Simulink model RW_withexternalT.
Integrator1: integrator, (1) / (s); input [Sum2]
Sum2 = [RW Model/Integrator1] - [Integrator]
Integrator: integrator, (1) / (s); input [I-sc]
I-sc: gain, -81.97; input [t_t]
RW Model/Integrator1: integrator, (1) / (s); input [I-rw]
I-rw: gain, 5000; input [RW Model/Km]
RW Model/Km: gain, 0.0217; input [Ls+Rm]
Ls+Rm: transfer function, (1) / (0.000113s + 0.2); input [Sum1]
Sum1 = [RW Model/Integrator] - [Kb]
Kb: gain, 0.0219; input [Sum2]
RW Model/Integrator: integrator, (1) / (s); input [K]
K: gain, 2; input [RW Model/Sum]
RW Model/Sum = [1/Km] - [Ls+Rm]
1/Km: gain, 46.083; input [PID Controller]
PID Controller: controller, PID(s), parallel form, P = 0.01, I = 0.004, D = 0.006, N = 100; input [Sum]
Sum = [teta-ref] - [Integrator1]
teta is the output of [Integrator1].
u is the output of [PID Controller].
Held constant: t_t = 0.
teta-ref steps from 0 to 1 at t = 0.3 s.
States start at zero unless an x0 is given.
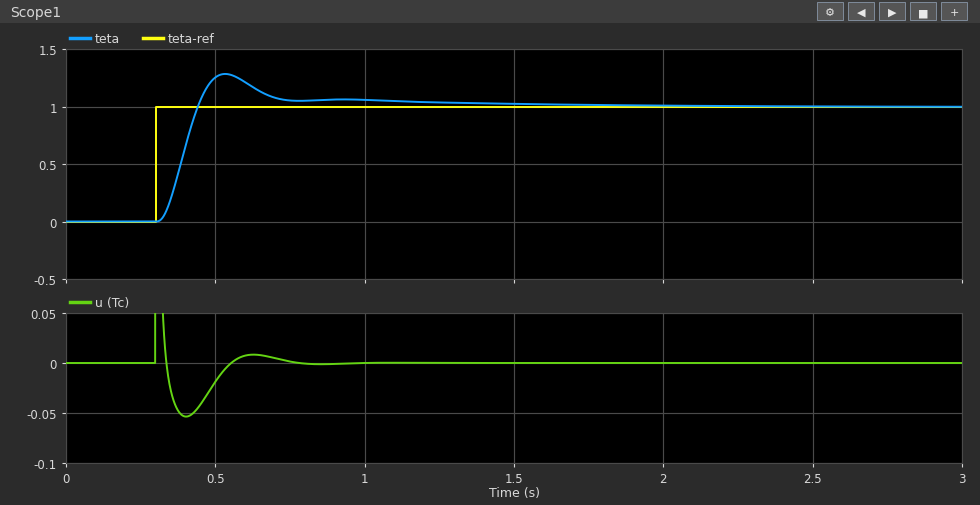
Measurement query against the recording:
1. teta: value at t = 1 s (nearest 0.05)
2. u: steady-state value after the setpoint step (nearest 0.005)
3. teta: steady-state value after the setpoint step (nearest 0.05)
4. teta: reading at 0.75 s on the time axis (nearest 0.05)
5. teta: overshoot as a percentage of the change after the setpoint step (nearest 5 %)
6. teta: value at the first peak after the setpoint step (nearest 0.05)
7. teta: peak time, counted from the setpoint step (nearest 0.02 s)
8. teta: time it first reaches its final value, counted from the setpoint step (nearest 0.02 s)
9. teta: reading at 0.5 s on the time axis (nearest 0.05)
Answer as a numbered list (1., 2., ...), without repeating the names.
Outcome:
1. 1.05
2. 0.000
3. 1.00
4. 1.05
5. 30 %
6. 1.30
7. 0.24 s
8. 0.14 s
9. 1.25
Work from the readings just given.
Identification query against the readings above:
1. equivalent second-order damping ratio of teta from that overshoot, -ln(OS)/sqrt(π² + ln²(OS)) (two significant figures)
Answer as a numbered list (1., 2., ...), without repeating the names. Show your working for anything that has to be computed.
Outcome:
1. ln(0.3) = -1.204; 1.204 / sqrt(9.870 + 1.450) = 0.36
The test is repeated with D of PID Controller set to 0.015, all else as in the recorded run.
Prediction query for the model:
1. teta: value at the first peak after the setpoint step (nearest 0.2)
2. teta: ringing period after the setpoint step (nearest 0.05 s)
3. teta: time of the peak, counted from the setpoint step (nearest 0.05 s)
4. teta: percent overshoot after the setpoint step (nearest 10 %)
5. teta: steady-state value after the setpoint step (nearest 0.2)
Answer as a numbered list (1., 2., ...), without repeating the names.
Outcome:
1. 1.4
2. 0.25 s
3. 0.15 s
4. 50 %
5. 1.0
